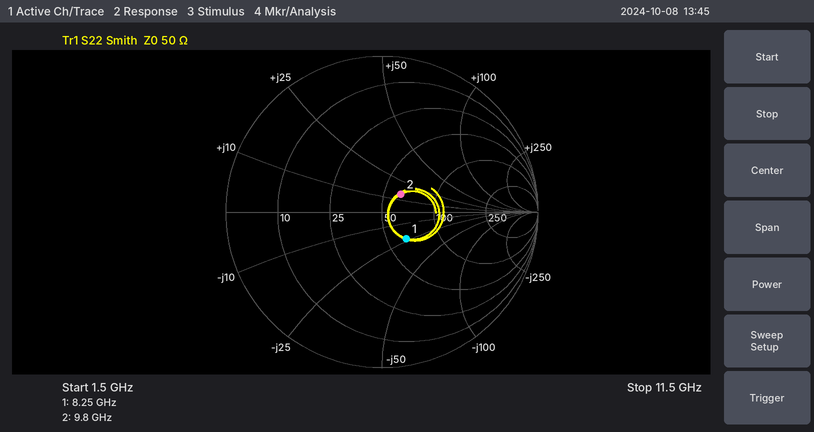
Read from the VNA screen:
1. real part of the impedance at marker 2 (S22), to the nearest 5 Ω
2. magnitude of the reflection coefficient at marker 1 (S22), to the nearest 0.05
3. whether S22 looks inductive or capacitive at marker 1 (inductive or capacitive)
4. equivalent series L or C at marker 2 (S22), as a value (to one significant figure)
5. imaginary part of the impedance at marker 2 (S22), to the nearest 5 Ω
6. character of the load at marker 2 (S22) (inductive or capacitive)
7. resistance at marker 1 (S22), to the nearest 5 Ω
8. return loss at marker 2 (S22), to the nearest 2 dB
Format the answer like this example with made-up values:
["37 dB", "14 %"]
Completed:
["60 Ω", "0.25", "capacitive", "200 pH", "+15 Ω", "inductive", "65 Ω", "16 dB"]
